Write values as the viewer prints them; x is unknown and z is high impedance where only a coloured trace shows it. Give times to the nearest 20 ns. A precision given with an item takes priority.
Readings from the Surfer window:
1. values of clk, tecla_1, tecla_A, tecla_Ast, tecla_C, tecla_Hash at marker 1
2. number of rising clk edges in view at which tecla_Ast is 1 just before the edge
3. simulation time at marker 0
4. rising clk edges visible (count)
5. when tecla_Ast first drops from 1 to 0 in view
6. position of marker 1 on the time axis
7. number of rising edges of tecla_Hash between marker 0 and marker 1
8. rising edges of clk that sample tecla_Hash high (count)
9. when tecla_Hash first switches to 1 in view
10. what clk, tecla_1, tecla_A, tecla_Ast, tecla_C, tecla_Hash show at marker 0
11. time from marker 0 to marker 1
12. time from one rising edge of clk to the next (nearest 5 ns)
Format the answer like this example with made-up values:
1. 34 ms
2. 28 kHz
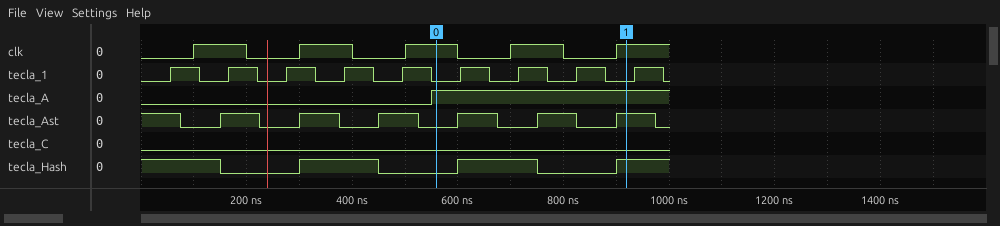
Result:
1. clk=1, tecla_1=0, tecla_A=1, tecla_Ast=1, tecla_C=0, tecla_Hash=1
2. 1
3. 560 ns
4. 5
5. 80 ns
6. 920 ns
7. 2
8. 2
9. 300 ns
10. clk=1, tecla_1=0, tecla_A=1, tecla_Ast=0, tecla_C=0, tecla_Hash=0
11. 360 ns
12. 200 ns
